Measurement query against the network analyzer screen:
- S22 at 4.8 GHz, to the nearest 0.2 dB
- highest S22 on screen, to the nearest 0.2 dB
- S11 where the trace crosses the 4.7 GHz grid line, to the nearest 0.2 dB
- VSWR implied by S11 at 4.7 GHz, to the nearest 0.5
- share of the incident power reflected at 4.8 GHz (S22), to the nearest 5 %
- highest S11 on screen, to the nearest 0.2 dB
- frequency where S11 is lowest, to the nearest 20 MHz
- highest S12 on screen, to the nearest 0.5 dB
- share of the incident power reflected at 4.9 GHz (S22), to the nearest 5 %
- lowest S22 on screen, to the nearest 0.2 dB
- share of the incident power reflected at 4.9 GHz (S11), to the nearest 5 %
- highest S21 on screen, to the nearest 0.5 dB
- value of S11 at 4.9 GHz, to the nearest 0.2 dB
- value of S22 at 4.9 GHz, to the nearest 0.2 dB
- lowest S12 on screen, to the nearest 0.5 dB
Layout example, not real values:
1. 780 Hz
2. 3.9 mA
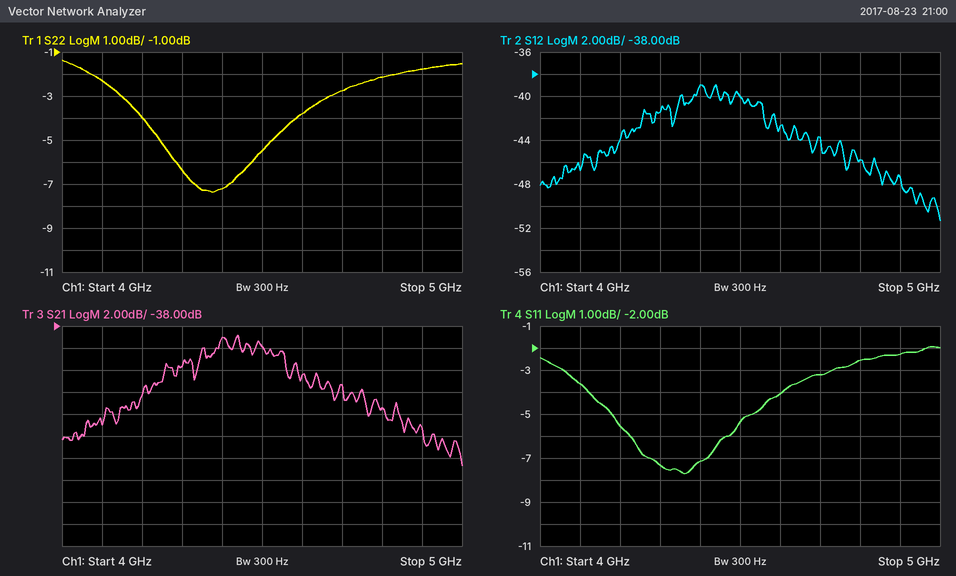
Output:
1. -2.2 dB
2. -1.4 dB
3. -3.2 dB
4. 5.5
5. 60 %
6. -2.0 dB
7. 4.36 GHz
8. -39.0 dB
9. 65 %
10. -7.4 dB
11. 60 %
12. -39.0 dB
13. -2.2 dB
14. -1.8 dB
15. -51.5 dB
